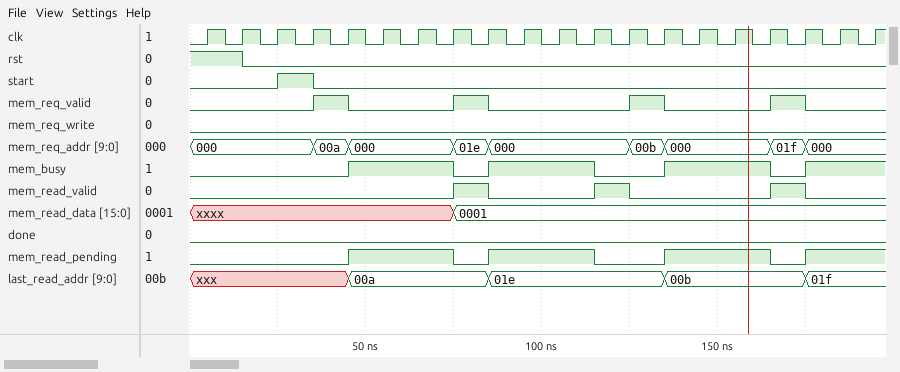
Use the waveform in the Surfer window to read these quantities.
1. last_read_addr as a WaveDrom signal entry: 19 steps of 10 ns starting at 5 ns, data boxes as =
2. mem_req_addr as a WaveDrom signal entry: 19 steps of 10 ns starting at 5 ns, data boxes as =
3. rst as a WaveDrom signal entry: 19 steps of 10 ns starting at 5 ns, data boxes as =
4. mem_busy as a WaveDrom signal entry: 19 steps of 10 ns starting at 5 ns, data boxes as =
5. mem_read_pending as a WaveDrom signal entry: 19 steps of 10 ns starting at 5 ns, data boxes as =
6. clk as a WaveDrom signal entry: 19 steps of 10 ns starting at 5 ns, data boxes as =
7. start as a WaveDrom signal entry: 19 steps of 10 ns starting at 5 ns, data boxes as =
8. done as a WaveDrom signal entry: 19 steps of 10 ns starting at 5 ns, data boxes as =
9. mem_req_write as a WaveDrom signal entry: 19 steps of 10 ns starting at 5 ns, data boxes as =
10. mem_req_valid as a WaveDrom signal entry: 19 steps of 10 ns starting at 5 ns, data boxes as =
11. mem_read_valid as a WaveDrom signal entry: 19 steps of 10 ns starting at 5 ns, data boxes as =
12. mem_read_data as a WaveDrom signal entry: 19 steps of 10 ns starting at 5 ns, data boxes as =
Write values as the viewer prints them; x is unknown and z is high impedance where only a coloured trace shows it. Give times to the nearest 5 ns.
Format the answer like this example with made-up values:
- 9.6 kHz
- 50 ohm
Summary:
- {name: 'last_read_addr', wave: 'x...=...=....=...=.', data: '00a 01e 00b 01f'}
- {name: 'mem_req_addr', wave: '=..==..==...==..==.', data: '000 00a 000 01e 000 00b 000 01f 000'}
- {name: 'rst', wave: '10.................'}
- {name: 'mem_busy', wave: '0...1..01..0.1..01.'}
- {name: 'mem_read_pending', wave: '0...1..01..0.1..01.'}
- {name: 'clk', wave: 'p..................'}
- {name: 'start', wave: '0.10...............'}
- {name: 'done', wave: '0..................'}
- {name: 'mem_req_write', wave: '0..................'}
- {name: 'mem_req_valid', wave: '0..10..10...10..10.'}
- {name: 'mem_read_valid', wave: '0......10..10...10.'}
- {name: 'mem_read_data', wave: 'x......=...........', data: '0001'}
